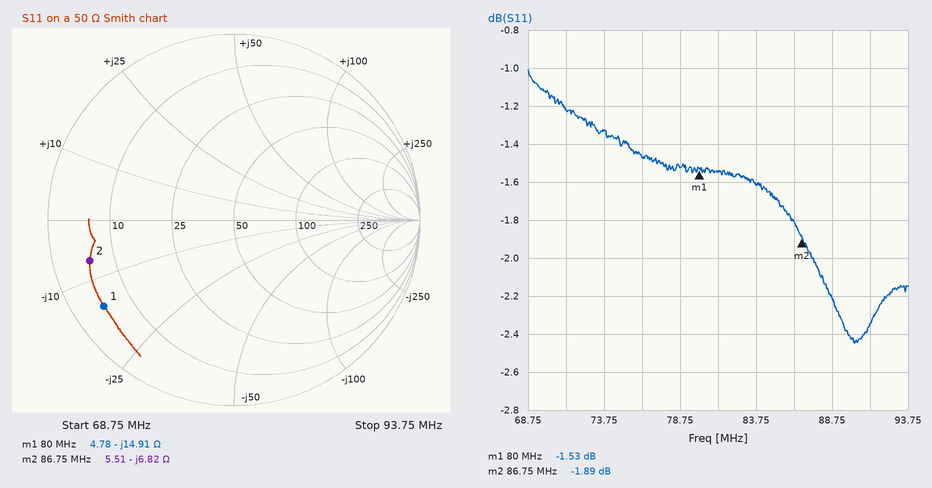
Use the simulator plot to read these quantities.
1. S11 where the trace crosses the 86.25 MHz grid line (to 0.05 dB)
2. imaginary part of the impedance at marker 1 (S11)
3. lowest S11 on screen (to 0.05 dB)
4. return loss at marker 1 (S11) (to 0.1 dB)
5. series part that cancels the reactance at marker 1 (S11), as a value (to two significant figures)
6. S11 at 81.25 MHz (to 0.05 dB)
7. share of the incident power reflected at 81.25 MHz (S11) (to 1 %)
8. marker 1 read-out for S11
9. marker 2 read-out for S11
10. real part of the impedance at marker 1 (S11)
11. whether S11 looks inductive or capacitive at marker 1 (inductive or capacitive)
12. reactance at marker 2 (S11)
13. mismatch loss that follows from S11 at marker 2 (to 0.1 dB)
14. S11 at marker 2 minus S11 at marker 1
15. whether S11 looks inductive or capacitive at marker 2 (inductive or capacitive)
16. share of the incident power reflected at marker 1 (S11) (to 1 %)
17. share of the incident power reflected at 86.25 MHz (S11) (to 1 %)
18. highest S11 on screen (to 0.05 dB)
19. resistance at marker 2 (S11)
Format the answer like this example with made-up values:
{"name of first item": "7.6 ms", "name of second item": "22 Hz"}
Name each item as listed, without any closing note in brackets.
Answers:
{"S11 where the trace crosses the 86.25 MHz grid line": "-1.80 dB", "imaginary part of the impedance at marker 1": "-14.91 Ω", "lowest S11 on screen": "-2.45 dB", "return loss at marker 1 (S11)": "1.5 dB", "series part that cancels the reactance at marker 1 (S11), as a value": "30 nH", "S11 at 81.25 MHz": "-1.55 dB", "share of the incident power reflected at 81.25 MHz (S11)": "70 %", "marker 1 read-out for S11": "-1.53 dB", "marker 2 read-out for S11": "-1.89 dB", "real part of the impedance at marker 1": "4.78 Ω", "whether S11 looks inductive or capacitive at marker 1": "capacitive", "reactance at marker 2": "-6.82 Ω", "mismatch loss that follows from S11 at marker 2": "4.5 dB", "S11 at marker 2 minus S11 at marker 1": "-0.36 dB", "whether S11 looks inductive or capacitive at marker 2": "capacitive", "share of the incident power reflected at marker 1 (S11)": "70 %", "share of the incident power reflected at 86.25 MHz (S11)": "66 %", "highest S11 on screen": "-1.00 dB", "resistance at marker 2": "5.51 Ω"}
